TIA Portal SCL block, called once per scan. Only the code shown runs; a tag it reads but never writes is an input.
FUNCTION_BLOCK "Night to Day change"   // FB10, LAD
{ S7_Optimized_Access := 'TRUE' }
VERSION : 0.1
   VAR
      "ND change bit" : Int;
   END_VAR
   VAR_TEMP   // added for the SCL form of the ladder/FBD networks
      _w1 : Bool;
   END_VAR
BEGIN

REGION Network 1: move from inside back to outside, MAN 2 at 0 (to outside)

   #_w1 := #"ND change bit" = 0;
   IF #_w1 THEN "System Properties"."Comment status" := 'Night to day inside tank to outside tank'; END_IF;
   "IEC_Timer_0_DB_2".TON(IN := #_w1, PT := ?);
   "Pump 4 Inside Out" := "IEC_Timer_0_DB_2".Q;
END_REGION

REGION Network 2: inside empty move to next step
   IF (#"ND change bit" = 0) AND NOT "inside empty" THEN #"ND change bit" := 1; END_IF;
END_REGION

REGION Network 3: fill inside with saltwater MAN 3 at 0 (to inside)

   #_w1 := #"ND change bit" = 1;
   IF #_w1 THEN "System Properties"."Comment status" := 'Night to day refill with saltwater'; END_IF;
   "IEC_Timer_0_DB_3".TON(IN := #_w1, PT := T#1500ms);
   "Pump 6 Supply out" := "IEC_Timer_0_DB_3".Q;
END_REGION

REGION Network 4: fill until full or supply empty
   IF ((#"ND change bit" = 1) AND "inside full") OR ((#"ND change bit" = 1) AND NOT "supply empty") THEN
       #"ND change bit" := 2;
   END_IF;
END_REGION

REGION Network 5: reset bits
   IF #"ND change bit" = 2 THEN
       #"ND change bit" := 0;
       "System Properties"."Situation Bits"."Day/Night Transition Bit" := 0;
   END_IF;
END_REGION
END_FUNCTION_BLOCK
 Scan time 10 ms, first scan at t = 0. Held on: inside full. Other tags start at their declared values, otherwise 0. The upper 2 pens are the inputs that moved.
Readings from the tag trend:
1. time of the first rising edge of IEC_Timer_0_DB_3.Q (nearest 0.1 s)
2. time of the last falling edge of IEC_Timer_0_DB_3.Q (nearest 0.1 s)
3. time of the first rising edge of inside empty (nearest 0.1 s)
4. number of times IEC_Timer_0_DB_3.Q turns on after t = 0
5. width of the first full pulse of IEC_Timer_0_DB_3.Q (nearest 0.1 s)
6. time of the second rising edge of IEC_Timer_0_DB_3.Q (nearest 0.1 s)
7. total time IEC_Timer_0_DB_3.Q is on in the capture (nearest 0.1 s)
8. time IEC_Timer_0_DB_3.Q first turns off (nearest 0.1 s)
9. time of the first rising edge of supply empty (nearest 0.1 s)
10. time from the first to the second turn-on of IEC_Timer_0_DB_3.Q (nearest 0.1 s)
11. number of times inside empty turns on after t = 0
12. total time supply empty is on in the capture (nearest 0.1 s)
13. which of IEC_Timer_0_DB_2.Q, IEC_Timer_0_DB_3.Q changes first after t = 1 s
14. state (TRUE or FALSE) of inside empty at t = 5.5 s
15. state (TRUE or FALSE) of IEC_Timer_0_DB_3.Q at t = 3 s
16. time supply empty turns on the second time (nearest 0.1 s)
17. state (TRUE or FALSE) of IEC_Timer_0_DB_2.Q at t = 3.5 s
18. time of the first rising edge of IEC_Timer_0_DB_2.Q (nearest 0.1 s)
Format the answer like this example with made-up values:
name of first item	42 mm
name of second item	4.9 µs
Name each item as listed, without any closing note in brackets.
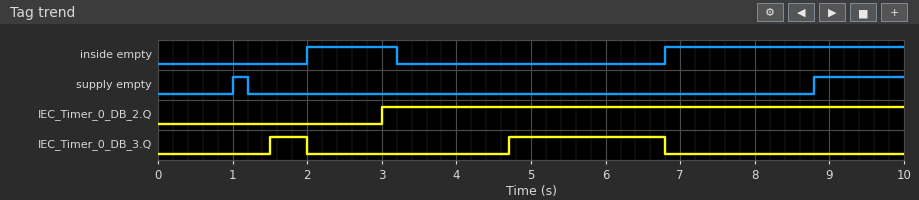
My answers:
time of the first rising edge of IEC_Timer_0_DB_3.Q	1.5 s
time of the last falling edge of IEC_Timer_0_DB_3.Q	6.8 s
time of the first rising edge of inside empty	2.0 s
number of times IEC_Timer_0_DB_3.Q turns on after t = 0	2
width of the first full pulse of IEC_Timer_0_DB_3.Q	0.5 s
time of the second rising edge of IEC_Timer_0_DB_3.Q	4.7 s
total time IEC_Timer_0_DB_3.Q is on in the capture	2.6 s
time IEC_Timer_0_DB_3.Q first turns off	2.0 s
time of the first rising edge of supply empty	1.0 s
time from the first to the second turn-on of IEC_Timer_0_DB_3.Q	3.2 s
number of times inside empty turns on after t = 0	2
total time supply empty is on in the capture	1.4 s
which of IEC_Timer_0_DB_2.Q, IEC_Timer_0_DB_3.Q changes first after t = 1 s	IEC_Timer_0_DB_3.Q
state (TRUE or FALSE) of inside empty at t = 5.5 s	FALSE
state (TRUE or FALSE) of IEC_Timer_0_DB_3.Q at t = 3 s	FALSE
time supply empty turns on the second time	8.8 s
state (TRUE or FALSE) of IEC_Timer_0_DB_2.Q at t = 3.5 s	TRUE
time of the first rising edge of IEC_Timer_0_DB_2.Q	3.0 s
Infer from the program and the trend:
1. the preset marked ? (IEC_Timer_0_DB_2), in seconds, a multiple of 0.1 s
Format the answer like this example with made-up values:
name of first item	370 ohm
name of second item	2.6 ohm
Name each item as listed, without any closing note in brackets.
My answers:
the preset marked ? (IEC_Timer_0_DB_2), in seconds, a multiple of 0.1 s	3.0 s
